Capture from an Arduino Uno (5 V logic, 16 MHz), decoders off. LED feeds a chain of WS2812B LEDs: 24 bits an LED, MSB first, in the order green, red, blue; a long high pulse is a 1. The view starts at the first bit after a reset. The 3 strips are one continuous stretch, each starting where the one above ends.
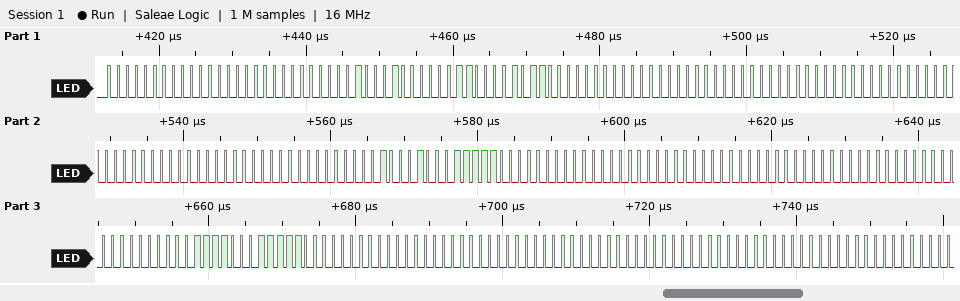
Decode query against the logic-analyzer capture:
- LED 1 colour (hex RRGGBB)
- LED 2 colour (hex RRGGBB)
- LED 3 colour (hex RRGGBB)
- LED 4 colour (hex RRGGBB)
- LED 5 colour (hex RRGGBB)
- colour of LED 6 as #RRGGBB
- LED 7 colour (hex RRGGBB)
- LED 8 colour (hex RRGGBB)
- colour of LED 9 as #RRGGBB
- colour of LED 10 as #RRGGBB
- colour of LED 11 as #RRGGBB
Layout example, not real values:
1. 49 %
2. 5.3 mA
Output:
1. #000000
2. #03110B
3. #000000
4. #000000
5. #000000
6. #1F1100
7. #000000
8. #000000
9. #1F0F00
10. #000000
11. #000000
